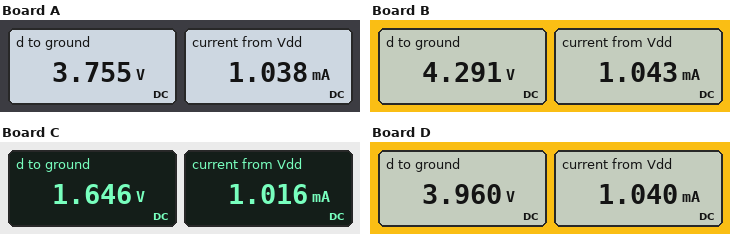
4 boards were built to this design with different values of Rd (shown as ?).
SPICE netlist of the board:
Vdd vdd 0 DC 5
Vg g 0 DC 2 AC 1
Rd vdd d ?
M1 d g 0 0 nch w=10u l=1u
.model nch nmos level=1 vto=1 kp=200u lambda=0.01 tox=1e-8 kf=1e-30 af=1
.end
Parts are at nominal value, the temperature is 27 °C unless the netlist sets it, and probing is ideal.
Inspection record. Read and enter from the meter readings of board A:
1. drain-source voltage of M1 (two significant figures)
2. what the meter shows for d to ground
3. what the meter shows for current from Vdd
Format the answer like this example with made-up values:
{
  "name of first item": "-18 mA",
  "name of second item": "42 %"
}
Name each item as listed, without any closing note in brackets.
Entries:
{
  "drain-source voltage of M1": "3.8 V",
  "what the meter shows for d to ground": "3.755 V",
  "what the meter shows for current from Vdd": "1.038 mA"
}
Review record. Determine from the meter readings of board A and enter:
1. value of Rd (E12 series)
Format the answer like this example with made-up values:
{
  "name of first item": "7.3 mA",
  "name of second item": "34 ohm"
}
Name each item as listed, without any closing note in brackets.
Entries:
{
  "value of Rd": "1.2 kΩ"
}
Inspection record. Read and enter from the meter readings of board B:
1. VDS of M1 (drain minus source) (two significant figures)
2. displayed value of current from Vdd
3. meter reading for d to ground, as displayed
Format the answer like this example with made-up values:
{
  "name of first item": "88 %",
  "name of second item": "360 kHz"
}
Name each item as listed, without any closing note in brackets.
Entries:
{
  "VDS of M1 (drain minus source)": "4.3 V",
  "displayed value of current from Vdd": "1.043 mA",
  "meter reading for d to ground, as displayed": "4.291 V"
}
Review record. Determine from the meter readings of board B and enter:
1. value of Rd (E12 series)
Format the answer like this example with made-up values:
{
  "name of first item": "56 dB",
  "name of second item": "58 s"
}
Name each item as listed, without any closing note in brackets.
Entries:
{
  "value of Rd": "680 Ω"
}
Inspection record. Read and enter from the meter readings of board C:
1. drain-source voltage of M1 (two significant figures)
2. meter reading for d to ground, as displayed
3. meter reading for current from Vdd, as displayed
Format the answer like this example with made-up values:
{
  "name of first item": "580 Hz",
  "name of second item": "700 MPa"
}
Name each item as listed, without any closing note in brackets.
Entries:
{
  "drain-source voltage of M1": "1.6 V",
  "meter reading for d to ground, as displayed": "1.646 V",
  "meter reading for current from Vdd, as displayed": "1.016 mA"
}
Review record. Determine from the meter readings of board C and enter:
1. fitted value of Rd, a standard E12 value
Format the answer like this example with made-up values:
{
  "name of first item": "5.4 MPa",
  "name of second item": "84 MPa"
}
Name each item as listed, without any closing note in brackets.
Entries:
{
  "fitted value of Rd, a standard E12 value": "3.3 kΩ"
}
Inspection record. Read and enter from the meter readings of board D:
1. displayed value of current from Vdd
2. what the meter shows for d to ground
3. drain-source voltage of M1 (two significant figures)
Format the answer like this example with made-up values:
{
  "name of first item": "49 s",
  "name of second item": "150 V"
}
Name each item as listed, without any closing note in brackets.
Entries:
{
  "displayed value of current from Vdd": "1.040 mA",
  "what the meter shows for d to ground": "3.960 V",
  "drain-source voltage of M1": "4.0 V"
}
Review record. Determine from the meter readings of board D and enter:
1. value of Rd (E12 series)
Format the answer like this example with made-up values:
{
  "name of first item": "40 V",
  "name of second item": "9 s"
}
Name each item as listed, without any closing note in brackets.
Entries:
{
  "value of Rd": "1 kΩ"
}
